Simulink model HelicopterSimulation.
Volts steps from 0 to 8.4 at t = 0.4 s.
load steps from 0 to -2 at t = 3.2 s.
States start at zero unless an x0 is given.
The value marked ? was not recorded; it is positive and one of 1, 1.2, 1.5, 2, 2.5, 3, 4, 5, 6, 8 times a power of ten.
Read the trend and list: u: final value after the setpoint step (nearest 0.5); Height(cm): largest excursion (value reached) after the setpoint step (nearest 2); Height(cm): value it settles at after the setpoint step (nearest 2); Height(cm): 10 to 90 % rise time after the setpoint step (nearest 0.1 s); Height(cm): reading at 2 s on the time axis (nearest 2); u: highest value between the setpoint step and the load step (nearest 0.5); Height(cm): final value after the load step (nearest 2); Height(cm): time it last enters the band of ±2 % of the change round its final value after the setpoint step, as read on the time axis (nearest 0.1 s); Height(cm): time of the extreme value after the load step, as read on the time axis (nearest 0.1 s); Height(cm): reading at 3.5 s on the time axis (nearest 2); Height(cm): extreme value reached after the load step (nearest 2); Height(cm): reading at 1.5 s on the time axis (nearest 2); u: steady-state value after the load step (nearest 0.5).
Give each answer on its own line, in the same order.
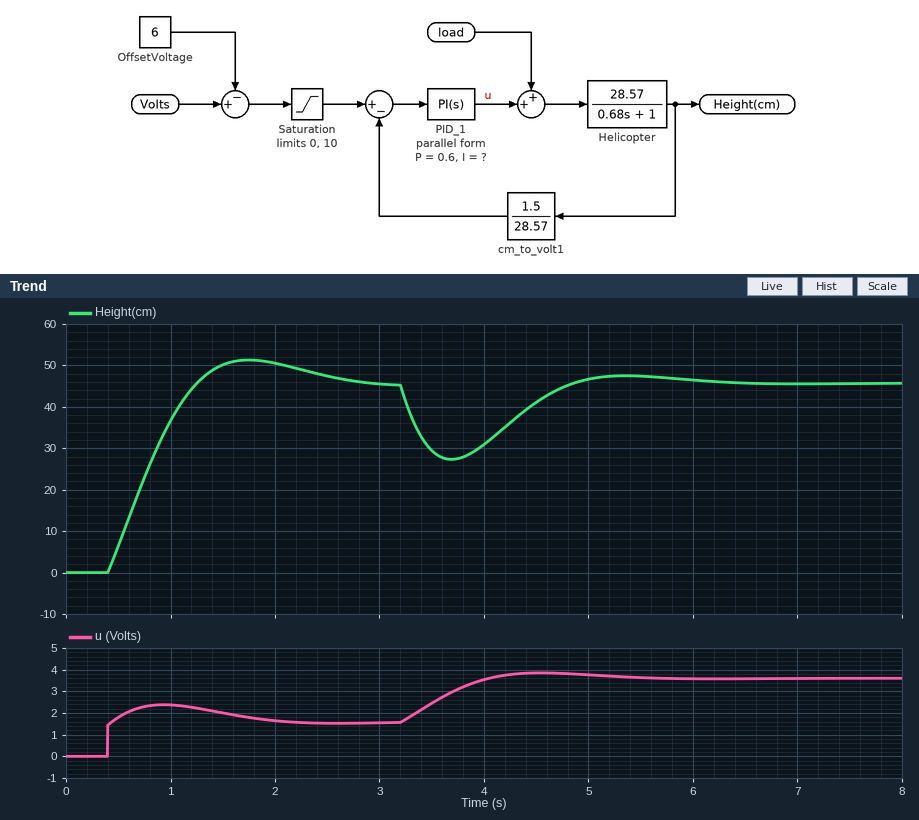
1.5
52
46
0.6 s
50
2.5
46
2.7 s
3.7 s
30
28
50
3.5
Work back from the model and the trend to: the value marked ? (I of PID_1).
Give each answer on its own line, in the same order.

2.5
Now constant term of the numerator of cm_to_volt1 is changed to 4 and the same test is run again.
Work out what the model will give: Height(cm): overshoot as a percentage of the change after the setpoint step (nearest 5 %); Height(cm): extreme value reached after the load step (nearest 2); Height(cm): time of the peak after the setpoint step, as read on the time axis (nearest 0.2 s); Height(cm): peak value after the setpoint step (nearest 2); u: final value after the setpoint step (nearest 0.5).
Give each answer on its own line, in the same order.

15 %
6
1.2 s
20
0.5
